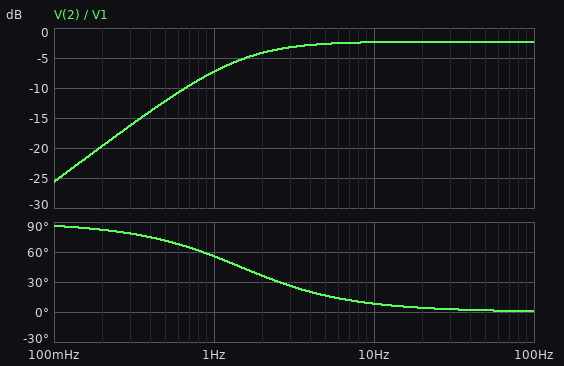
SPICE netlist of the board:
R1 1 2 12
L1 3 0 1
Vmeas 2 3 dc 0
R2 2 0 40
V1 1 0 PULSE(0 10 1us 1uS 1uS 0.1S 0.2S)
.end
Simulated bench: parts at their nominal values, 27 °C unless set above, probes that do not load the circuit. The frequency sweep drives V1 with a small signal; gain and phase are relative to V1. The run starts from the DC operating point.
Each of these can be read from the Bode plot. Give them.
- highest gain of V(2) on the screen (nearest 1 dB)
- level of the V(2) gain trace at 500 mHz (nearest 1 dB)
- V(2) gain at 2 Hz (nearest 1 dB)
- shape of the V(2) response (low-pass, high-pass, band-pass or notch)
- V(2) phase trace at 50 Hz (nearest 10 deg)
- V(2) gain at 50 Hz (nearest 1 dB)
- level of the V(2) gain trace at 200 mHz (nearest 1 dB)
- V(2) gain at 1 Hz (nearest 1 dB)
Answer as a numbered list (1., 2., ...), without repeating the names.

1. -2 dB
2. -12 dB
3. -4 dB
4. high-pass
5. 0 deg
6. -2 dB
7. -20 dB
8. -7 dB
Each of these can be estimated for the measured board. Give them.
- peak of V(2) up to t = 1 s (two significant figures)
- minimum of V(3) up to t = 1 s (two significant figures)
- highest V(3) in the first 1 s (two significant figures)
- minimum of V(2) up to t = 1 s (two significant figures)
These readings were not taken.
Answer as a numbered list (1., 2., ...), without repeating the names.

1. 7.7 V
2. -5.5 V
3. 7.7 V
4. -5.5 V
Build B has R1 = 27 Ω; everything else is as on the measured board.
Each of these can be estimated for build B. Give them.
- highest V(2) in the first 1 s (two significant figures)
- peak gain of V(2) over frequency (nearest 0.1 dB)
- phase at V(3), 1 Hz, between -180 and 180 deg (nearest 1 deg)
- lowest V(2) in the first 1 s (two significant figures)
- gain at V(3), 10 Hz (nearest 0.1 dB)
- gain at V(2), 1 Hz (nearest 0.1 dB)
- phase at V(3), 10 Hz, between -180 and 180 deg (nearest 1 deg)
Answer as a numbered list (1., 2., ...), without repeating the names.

1. 6.0 V
2. -4.5 dB
3. 69 deg
4. -5.0 V
5. -4.8 dB
6. -13.3 dB
7. 14 deg
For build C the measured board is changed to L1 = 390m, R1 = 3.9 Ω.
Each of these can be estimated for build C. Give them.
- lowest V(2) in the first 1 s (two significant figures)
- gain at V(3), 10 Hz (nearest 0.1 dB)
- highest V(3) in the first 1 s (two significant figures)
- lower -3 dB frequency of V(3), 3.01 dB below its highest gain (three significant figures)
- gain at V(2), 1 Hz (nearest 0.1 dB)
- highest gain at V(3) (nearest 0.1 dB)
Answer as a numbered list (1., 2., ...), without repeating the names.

1. -6.5 V
2. -0.9 dB
3. 9.1 V
4. 1.45 Hz
5. -5.7 dB
6. -0.8 dB
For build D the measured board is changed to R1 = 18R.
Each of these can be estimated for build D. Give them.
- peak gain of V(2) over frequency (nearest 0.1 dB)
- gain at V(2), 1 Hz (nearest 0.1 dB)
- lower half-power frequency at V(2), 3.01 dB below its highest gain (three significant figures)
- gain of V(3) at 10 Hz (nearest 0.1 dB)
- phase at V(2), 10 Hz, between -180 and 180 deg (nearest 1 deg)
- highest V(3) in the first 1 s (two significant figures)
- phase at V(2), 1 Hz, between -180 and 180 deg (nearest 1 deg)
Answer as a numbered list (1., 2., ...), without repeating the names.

1. -3.2 dB
2. -10.1 dB
3. 1.98 Hz
4. -3.4 dB
5. 11 deg
6. 6.9 V
7. 63 deg
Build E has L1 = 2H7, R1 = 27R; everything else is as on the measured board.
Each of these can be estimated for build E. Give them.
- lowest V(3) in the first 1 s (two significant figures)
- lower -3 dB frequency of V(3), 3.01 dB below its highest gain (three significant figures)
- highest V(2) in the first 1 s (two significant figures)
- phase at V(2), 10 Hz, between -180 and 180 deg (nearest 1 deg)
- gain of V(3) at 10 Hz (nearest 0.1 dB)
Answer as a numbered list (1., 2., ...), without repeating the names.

1. -3.8 V
2. 950 mHz
3. 6.0 V
4. 5 deg
5. -4.5 dB
